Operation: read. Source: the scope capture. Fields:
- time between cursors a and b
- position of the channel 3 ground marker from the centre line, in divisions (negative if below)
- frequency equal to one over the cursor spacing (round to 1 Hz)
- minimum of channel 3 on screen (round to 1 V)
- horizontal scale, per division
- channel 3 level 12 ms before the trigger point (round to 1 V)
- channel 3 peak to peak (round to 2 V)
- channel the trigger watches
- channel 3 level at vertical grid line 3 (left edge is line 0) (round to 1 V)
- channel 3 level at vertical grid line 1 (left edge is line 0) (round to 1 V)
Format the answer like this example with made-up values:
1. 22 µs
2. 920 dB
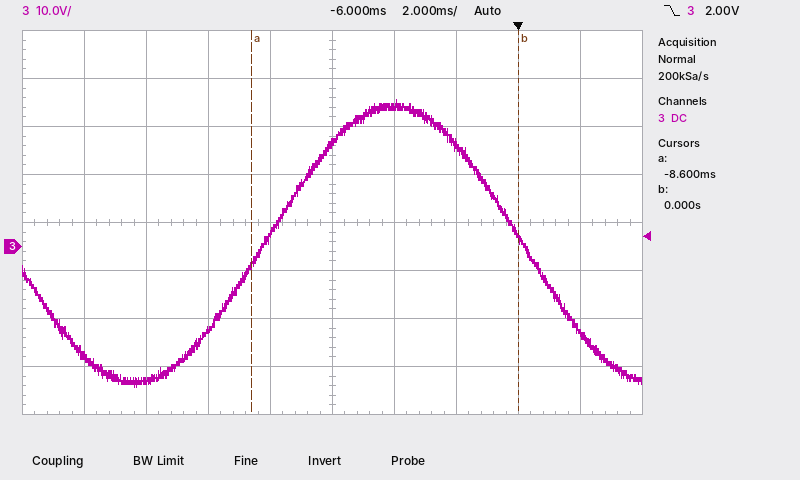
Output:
1. 8.6 ms
2. -0.5 div
3. 116 Hz
4. -29 V
5. 2 ms
6. -28 V
7. 60 V
8. channel 3
9. -18 V
10. -23 V
